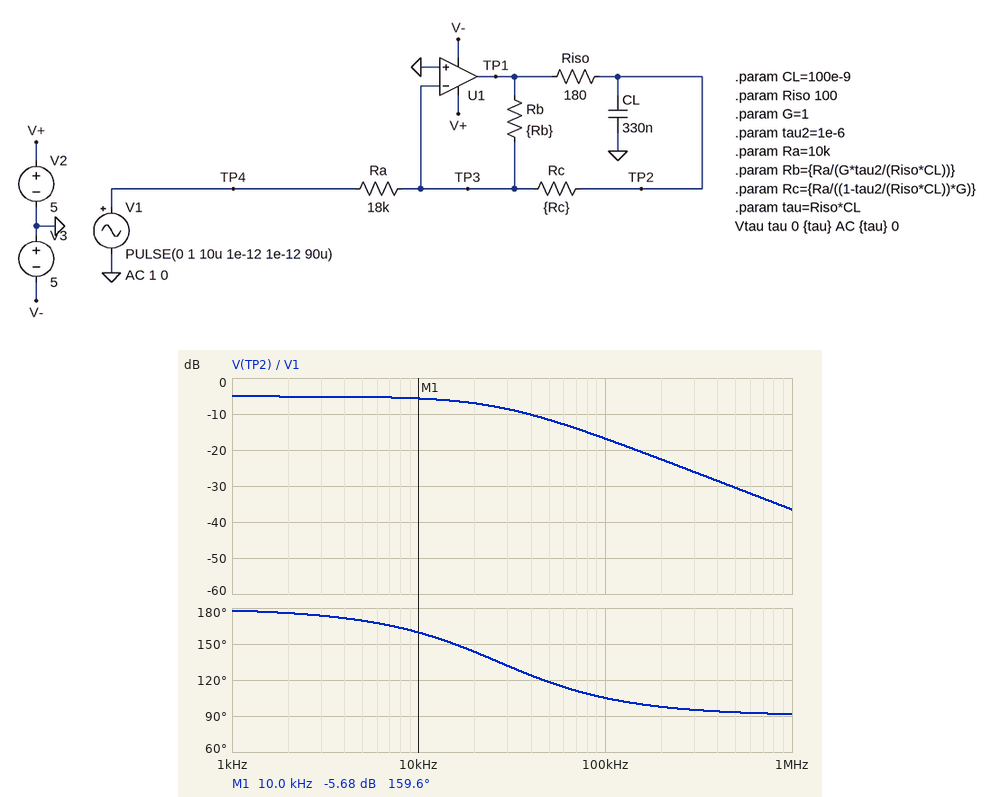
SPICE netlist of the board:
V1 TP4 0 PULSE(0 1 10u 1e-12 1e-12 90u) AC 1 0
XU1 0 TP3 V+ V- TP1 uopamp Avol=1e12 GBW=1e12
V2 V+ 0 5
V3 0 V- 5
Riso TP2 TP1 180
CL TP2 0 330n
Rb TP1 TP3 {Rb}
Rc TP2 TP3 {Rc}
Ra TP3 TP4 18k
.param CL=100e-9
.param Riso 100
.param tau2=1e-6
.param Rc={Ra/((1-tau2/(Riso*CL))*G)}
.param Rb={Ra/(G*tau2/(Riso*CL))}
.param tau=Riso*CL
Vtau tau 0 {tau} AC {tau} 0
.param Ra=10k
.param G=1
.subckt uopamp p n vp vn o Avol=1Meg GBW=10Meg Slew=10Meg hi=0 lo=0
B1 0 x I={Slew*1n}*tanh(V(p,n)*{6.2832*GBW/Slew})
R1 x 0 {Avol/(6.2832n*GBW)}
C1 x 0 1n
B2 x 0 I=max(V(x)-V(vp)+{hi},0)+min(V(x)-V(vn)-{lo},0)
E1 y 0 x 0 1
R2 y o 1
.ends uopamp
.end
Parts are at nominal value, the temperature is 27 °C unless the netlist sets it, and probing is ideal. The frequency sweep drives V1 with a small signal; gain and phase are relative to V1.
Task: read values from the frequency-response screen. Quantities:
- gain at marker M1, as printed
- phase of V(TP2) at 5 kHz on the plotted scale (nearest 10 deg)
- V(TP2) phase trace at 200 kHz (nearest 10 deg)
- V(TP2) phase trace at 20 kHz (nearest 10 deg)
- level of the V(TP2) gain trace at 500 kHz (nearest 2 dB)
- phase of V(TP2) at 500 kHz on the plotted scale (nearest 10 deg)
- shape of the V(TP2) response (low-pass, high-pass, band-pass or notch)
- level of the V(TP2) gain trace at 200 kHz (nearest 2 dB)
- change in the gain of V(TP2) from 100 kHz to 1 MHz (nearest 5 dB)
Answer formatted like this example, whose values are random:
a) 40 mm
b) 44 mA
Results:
a) -5.68 dB
b) 170 deg
c) 100 deg
d) 140 deg
e) -30 dB
f) 90 deg
g) low-pass
h) -22 dB
i) -20 dB
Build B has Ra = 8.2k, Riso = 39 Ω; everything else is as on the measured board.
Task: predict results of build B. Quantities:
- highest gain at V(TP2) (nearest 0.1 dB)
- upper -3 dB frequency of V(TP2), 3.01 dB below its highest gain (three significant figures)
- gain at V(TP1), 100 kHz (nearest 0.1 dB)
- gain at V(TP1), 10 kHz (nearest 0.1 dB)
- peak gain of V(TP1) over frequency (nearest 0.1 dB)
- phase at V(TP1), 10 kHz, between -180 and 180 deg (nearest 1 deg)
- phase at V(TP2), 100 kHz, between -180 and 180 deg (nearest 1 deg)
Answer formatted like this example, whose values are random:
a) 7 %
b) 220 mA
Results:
a) 1.7 dB
b) 124 kHz
c) 17.8 dB
d) 3.9 dB
e) 21.7 dB
f) -146 deg
g) 141 deg
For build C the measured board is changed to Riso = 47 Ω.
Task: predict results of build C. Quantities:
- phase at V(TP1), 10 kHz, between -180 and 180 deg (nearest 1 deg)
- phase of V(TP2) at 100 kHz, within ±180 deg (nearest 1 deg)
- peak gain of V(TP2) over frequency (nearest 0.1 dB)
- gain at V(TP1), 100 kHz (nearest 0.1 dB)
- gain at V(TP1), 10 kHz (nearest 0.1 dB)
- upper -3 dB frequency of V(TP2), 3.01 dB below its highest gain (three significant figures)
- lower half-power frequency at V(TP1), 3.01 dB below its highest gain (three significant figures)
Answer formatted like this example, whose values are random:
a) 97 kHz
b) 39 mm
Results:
a) -141 deg
b) 136 deg
c) -5.1 dB
d) 11.8 dB
e) -2.2 dB
f) 103 kHz
g) 102 kHz
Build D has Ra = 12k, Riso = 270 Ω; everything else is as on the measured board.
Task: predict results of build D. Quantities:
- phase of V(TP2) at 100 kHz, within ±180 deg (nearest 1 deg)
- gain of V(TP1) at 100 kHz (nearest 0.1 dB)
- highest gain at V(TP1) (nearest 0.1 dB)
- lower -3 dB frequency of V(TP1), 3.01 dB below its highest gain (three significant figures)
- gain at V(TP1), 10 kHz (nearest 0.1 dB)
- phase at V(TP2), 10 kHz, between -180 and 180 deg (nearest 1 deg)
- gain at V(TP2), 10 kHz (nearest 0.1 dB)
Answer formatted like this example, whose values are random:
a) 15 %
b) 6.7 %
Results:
a) 100 deg
b) 18.3 dB
c) 18.4 dB
d) 17.7 kHz
e) 12.3 dB
f) 151 deg
g) -2.8 dB
